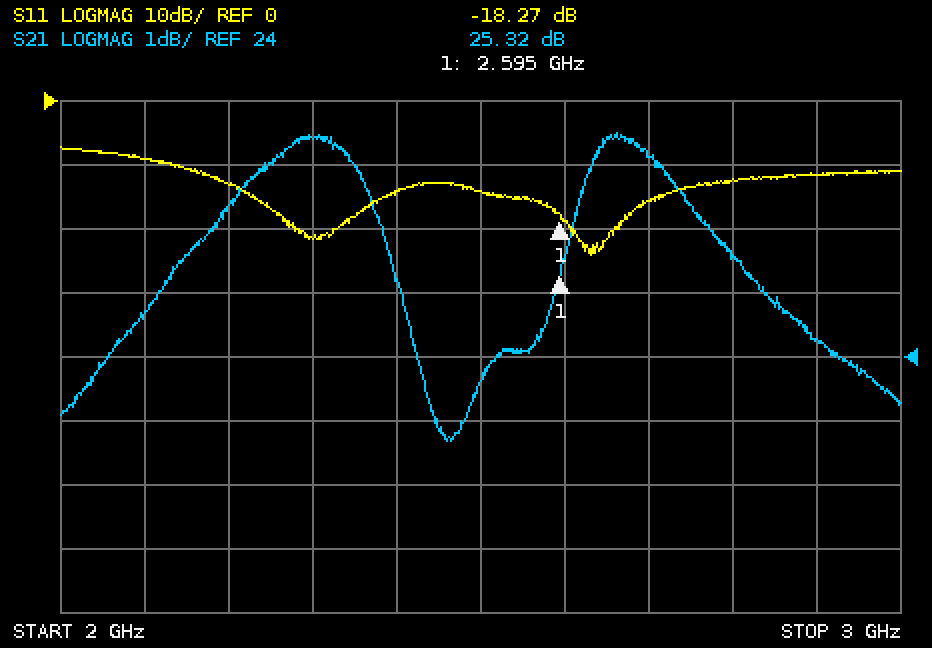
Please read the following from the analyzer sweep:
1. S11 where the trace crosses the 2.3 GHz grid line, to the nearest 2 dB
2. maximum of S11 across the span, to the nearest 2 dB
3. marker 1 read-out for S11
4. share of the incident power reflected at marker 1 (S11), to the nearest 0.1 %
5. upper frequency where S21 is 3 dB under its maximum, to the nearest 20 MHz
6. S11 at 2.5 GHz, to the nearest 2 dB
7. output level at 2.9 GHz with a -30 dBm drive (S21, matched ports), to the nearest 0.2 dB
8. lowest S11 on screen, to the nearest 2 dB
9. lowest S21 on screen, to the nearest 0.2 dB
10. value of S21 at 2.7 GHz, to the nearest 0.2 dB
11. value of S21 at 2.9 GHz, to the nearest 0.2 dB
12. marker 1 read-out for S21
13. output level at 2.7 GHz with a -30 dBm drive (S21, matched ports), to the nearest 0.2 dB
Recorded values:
-22 dB
-8 dB
-18.27 dB
1.5 %
2.88 GHz
-14 dB
-5.8 dBm
-24 dB
22.6 dB
27.2 dB
24.2 dB
25.32 dB
-2.8 dBm
